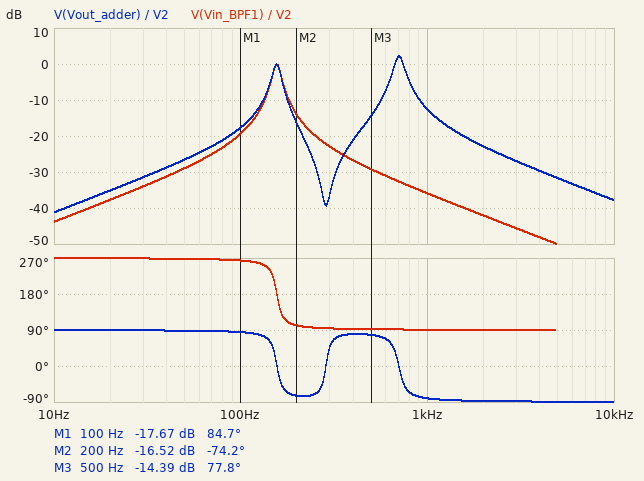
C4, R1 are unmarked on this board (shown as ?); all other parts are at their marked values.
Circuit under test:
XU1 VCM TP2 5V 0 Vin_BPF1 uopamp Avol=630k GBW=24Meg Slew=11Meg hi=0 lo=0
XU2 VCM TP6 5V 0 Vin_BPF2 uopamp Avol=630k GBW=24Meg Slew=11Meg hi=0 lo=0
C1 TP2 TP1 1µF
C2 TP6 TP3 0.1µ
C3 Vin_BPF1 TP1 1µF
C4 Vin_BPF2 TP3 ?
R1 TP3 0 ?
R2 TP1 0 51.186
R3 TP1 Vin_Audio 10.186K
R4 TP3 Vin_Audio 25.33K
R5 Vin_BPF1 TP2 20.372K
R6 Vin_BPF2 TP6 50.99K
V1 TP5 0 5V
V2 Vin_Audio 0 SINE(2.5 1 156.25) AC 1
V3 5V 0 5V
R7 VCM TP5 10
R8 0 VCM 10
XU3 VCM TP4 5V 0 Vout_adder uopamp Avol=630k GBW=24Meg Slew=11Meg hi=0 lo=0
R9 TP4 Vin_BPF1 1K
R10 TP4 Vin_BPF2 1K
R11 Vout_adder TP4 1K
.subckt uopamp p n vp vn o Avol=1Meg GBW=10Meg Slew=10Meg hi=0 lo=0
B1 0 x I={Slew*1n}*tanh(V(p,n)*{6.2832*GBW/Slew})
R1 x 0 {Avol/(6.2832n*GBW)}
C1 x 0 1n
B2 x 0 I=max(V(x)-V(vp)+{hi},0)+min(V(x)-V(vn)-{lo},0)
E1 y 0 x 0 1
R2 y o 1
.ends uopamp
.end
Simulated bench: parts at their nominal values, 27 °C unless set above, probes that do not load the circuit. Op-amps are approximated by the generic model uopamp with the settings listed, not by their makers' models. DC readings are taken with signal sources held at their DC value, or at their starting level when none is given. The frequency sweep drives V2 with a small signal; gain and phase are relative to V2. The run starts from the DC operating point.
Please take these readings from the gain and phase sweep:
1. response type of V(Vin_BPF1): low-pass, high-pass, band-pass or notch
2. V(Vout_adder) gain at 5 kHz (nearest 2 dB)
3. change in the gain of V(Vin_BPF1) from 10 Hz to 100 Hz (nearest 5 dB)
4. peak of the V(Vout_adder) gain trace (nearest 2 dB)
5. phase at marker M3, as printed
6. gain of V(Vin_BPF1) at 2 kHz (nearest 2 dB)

band-pass
-32 dB
25 dB
2 dB
77.8 deg
-42 dB
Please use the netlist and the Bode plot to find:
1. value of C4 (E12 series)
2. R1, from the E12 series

56 nF
180 Ω
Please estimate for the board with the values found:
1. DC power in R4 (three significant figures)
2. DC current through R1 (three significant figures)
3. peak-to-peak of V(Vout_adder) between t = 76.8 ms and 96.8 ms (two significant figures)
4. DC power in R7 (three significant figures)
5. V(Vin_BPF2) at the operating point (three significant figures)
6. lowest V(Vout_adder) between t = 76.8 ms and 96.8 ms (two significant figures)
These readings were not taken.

243 µW
98.0 µA
2.0 V
625 mW
2.50 V
1.5 V
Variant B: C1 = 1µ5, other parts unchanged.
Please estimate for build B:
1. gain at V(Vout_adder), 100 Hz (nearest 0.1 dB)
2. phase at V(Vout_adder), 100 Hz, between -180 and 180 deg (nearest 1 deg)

-11.5 dB
79 deg
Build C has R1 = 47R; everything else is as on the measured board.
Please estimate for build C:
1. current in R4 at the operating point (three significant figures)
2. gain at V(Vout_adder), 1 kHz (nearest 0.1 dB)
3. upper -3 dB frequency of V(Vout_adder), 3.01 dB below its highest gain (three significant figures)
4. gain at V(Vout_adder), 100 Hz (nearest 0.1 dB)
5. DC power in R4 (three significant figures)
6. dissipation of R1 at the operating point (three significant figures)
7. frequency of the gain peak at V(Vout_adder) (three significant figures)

98.5 µA
-19.2 dB
1.42 kHz
-18.9 dB
246 µW
456 nW
1.37 kHz
